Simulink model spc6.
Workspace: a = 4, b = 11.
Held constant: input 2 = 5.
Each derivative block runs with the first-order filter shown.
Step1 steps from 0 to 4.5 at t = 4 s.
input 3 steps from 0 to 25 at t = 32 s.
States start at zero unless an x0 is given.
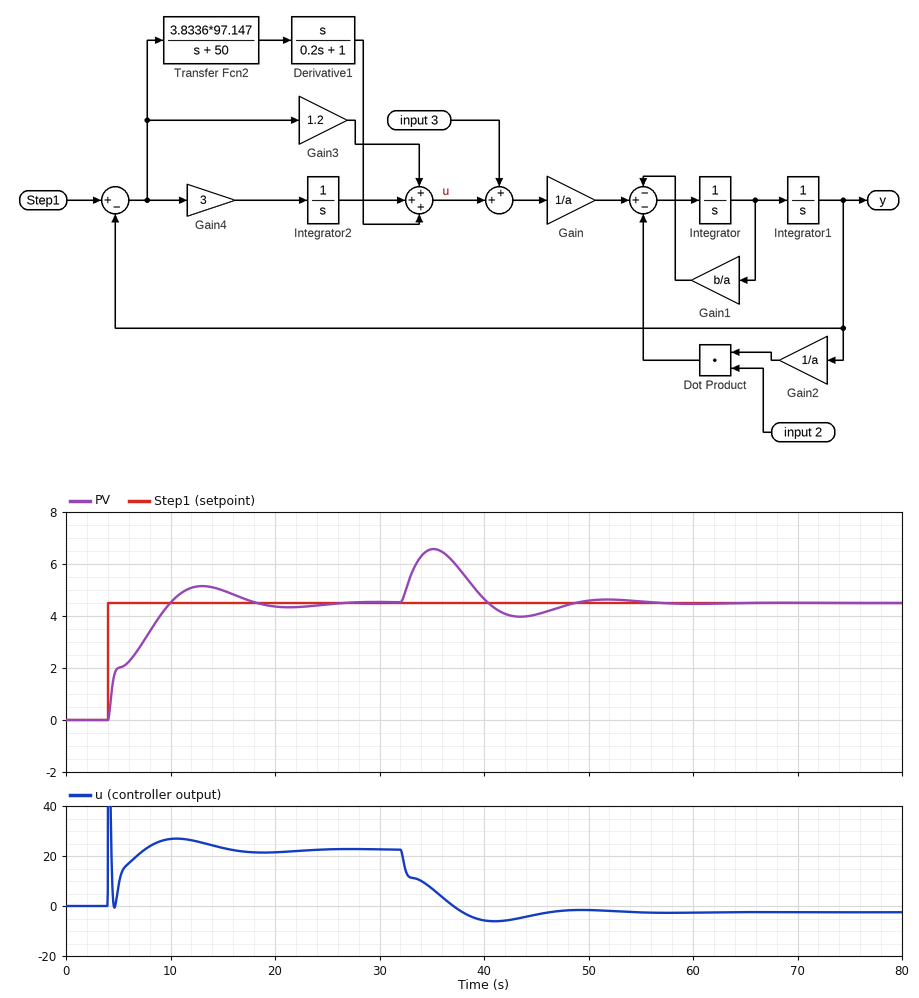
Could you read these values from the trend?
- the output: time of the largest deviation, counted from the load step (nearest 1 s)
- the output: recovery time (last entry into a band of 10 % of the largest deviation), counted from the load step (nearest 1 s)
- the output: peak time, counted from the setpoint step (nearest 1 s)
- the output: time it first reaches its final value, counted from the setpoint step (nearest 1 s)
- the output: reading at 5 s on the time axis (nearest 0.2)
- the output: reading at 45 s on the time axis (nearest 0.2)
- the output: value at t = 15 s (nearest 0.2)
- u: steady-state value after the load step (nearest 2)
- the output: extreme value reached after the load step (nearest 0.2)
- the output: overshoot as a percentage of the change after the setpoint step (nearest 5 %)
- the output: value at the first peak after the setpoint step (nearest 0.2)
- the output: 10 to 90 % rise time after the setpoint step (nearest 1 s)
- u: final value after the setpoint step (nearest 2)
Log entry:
3 s
15 s
9 s
6 s
2.0
4.0
5.0
-2
6.6
15 %
5.2
5 s
22
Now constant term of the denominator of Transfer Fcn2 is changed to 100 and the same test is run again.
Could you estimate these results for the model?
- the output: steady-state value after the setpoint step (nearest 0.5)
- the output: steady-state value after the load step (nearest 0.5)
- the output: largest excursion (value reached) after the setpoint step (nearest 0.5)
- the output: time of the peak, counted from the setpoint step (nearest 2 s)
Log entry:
4.5
4.5
5.0
8 s
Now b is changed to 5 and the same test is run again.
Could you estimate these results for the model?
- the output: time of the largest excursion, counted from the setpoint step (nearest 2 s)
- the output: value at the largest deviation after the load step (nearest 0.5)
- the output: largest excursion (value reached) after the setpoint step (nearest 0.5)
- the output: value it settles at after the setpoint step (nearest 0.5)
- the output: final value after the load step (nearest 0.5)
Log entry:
8 s
7.0
5.0
4.5
4.5
